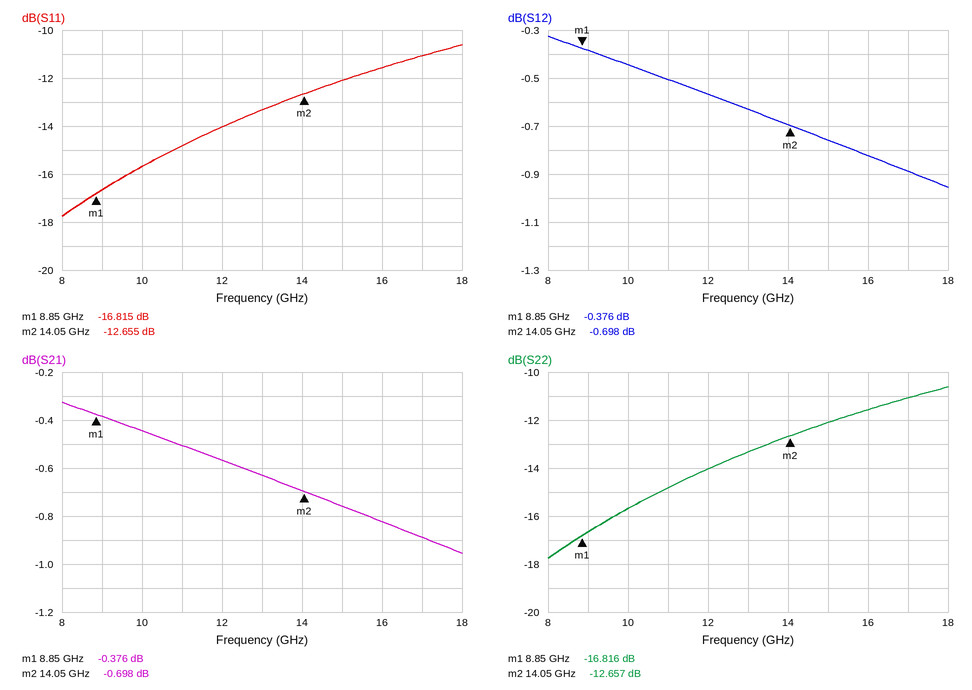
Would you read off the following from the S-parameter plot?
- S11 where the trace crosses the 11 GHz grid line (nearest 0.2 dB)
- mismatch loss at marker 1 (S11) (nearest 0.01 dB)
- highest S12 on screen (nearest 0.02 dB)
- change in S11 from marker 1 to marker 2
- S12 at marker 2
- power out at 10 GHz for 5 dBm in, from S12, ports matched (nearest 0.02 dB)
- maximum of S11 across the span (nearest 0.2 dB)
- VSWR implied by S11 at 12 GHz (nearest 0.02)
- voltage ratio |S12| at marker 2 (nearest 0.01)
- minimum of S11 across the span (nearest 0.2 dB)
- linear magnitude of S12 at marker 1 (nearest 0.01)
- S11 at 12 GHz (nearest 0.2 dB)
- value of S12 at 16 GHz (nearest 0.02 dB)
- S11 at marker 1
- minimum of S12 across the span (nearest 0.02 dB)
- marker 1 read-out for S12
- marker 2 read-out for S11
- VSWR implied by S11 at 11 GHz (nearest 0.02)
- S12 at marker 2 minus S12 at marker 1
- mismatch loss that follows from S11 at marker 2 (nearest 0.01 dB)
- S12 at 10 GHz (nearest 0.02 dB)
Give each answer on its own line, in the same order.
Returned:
-14.8 dB
0.09 dB
-0.32 dB
4.160 dB
-0.698 dB
4.56 dBm
-10.6 dB
1.50
0.92
-17.8 dB
0.96
-14.0 dB
-0.82 dB
-16.815 dB
-0.96 dB
-0.376 dB
-12.655 dB
1.44
-0.322 dB
0.24 dB
-0.44 dB
